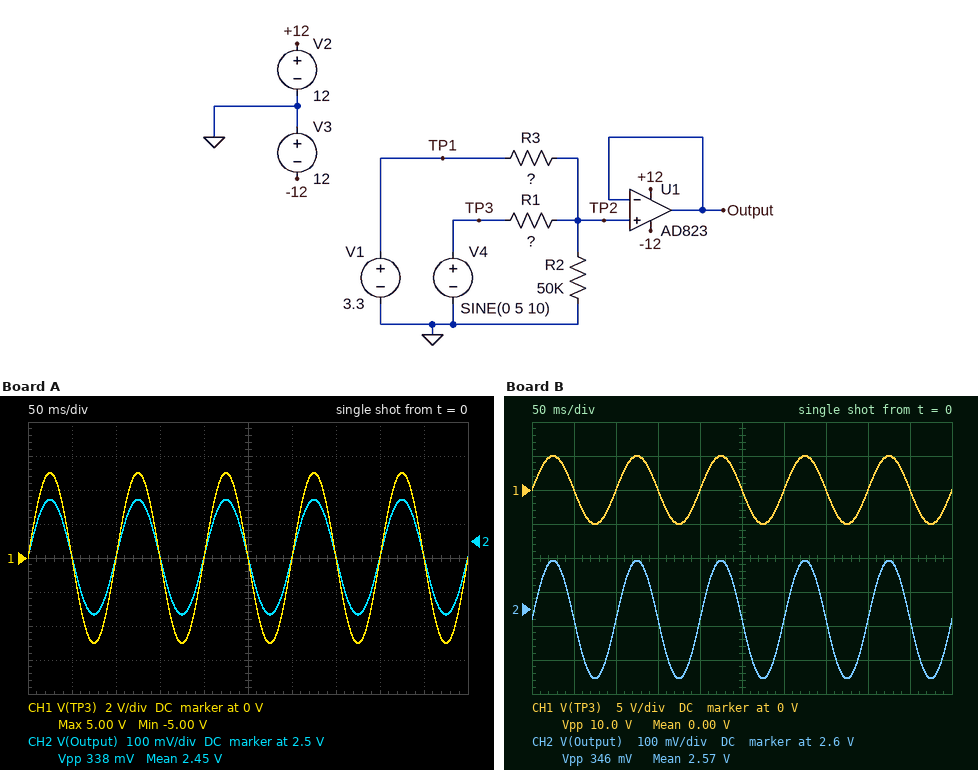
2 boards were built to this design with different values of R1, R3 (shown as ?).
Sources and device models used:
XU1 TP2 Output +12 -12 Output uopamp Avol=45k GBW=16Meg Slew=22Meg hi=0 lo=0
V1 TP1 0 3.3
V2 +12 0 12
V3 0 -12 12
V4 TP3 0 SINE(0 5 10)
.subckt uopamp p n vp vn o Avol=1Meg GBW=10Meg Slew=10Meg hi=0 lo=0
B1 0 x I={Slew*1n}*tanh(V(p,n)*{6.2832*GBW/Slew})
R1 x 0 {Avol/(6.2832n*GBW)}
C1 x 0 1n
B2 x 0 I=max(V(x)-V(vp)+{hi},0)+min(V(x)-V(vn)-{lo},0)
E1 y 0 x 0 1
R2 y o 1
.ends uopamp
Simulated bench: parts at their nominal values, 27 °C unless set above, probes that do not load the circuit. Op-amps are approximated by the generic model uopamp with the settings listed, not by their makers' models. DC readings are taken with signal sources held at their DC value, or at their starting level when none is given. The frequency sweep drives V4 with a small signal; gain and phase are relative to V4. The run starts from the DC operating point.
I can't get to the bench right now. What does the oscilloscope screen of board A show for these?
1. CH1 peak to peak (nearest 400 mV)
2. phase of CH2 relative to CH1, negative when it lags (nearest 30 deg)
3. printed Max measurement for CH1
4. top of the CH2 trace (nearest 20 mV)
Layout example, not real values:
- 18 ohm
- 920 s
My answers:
- 10.0 V
- 0 deg
- 5.00 V
- 2.62 V
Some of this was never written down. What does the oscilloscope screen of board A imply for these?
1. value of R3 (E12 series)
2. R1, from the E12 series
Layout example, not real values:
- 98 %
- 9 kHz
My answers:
- 15 kΩ
- 330 kΩ
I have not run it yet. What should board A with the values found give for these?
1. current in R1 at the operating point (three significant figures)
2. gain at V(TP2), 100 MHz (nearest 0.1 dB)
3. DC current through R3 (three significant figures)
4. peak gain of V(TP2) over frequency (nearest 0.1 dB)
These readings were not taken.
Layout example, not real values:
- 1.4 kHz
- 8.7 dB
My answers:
- 7.43 µA
- -29.4 dB
- 56.5 µA
- -29.4 dB
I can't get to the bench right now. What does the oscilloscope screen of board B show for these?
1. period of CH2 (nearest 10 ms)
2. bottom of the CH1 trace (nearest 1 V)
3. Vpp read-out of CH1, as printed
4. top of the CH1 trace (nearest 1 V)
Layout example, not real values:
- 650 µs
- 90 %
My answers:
- 100 ms
- -5 V
- 10.0 V
- 5 V
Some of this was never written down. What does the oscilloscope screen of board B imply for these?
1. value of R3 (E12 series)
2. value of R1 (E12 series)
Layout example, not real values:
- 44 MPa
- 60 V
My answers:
- 12 kΩ
- 270 kΩ
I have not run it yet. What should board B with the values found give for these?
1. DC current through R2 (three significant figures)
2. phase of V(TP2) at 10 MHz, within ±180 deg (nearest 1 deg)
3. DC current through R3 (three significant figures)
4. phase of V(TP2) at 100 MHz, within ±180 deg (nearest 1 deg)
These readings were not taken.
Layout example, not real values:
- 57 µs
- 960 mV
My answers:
- 51.4 µA
- 0 deg
- 60.9 µA
- 0 deg
